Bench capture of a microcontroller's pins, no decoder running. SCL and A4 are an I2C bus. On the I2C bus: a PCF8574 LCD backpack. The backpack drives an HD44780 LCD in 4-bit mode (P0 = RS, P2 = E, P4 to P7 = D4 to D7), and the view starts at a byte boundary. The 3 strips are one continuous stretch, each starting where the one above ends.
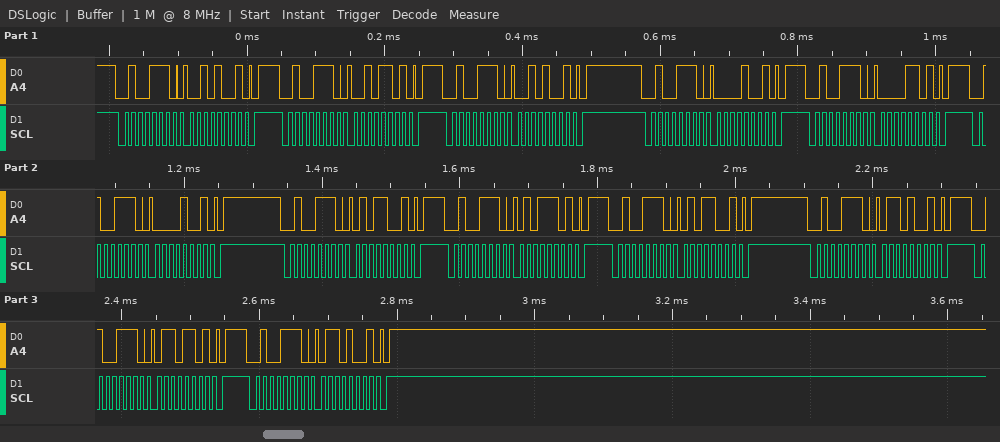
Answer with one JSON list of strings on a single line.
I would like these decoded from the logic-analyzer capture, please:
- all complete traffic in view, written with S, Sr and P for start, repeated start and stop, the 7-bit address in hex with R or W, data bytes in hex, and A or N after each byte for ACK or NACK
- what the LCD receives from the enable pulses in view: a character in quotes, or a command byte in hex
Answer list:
["S 27W A 29 A P S 27W A 2D A P S 27W A 29 A P S 27W A 09 A P S 27W A 0D A P S 27W A 09 A P S 27W A 59 A P S 27W A 5D A P S 27W A 59 A P S 27W A 69 A P S 27W A 6D A P S 27W A 69 A P", "' ' 'V'"]
